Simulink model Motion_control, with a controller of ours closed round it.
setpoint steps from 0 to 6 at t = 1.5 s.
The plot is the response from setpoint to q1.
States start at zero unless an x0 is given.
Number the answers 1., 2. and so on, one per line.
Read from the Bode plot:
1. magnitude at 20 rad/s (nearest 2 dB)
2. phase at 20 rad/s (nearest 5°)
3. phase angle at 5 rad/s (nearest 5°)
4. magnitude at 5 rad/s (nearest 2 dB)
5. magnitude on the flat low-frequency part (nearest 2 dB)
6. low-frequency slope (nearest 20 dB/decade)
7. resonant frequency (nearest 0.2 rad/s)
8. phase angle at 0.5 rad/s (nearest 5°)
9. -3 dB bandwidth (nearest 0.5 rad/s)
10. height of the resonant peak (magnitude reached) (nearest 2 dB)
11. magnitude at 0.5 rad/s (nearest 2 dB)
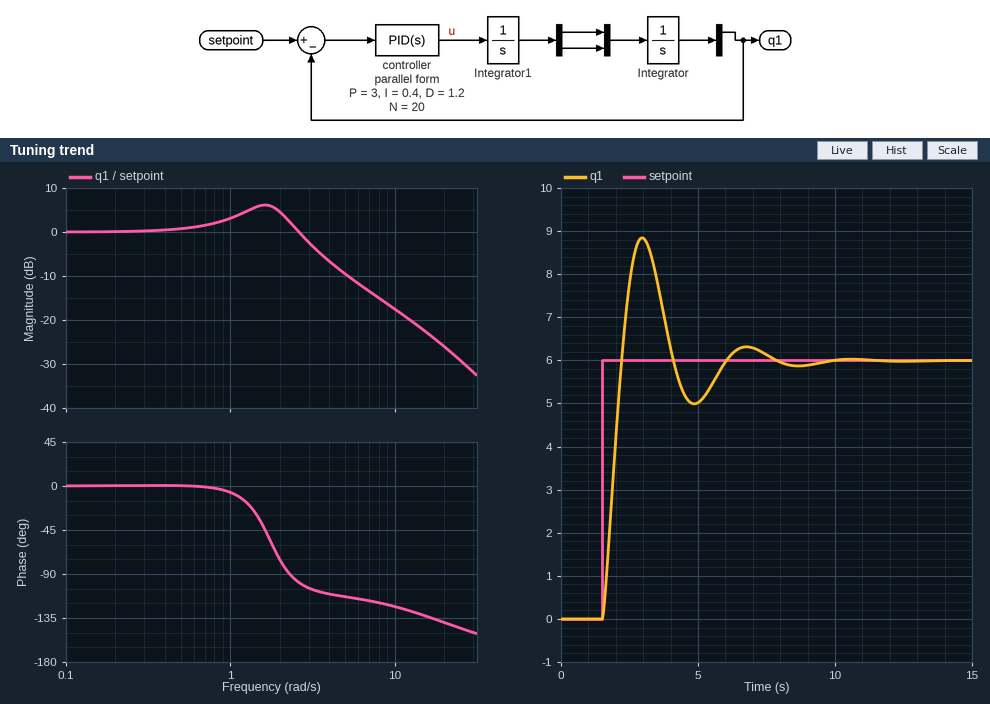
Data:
1. -26 dB
2. -140°
3. -115°
4. -10 dB
5. 0 dB
6. 0 dB/decade
7. 1.6 rad/s
8. 0°
9. 3.0 rad/s
10. 6 dB
11. 0 dB
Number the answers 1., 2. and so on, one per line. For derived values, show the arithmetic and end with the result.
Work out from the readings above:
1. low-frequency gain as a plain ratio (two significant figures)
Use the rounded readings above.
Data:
1. 10^(0 / 20) = 1.0
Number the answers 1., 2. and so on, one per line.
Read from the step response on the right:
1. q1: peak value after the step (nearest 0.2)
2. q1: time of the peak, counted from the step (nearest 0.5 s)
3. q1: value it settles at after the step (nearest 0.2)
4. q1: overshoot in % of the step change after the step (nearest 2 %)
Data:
1. 8.8
2. 1.5 s
3. 6.0
4. 48 %
